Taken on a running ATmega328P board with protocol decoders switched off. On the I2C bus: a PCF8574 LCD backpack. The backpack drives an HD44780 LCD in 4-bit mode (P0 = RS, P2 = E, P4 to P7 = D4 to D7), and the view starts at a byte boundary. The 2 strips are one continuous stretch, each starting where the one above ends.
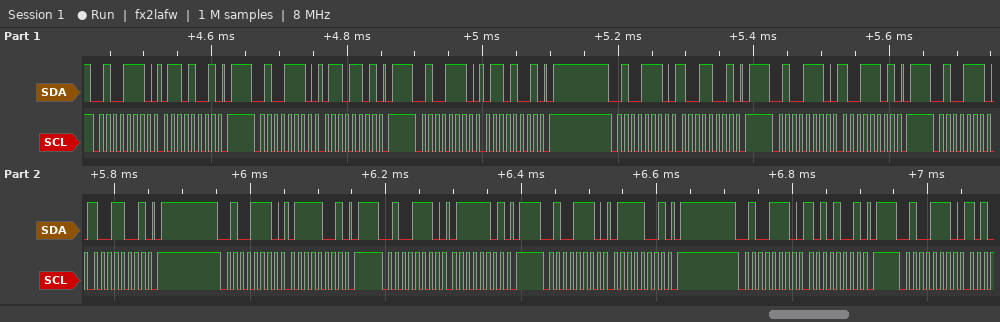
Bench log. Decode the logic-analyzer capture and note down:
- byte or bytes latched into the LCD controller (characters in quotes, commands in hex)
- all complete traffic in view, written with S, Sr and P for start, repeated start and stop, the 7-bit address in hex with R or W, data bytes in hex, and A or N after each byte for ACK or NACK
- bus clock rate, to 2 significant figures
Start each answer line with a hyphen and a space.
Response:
- 'i'
- S 27W A 69 A P S 27W A 6D A P S 27W A 69 A P S 27W A 99 A P S 27W A 9D A P S 27W A 99 A P S 27W A 79 A P S 27W A 7D A P S 27W A 79 A P S 27W A A9 A P S 27W A
- 100 kHz
